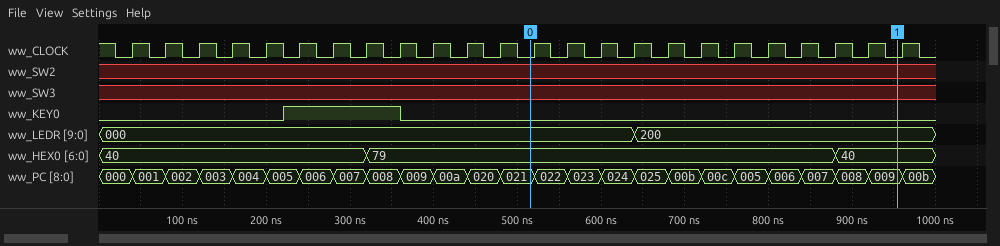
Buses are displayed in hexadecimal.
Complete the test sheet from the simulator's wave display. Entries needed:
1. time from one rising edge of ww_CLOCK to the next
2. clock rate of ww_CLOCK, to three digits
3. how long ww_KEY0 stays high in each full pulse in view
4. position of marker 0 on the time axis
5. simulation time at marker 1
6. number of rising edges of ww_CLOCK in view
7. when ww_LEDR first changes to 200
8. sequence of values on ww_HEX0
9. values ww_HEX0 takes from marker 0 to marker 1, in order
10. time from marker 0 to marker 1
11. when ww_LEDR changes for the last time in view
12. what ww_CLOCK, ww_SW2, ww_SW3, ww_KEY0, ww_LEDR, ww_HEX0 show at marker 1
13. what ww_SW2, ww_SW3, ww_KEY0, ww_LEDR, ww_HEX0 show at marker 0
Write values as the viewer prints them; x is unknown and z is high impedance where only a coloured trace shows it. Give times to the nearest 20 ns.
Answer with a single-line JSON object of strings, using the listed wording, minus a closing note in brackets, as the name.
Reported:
{"time from one rising edge of ww_CLOCK to the next": "40 ns", "clock rate of ww_CLOCK, to three digits": "25.0 MHz", "how long ww_KEY0 stays high in each full pulse in view": "140 ns", "position of marker 0 on the time axis": "520 ns", "simulation time at marker 1": "960 ns", "number of rising edges of ww_CLOCK in view": "24", "when ww_LEDR first changes to 200": "640 ns", "sequence of values on ww_HEX0": "40, 79, 40", "values ww_HEX0 takes from marker 0 to marker 1, in order": "79, 40", "time from marker 0 to marker 1": "440 ns", "when ww_LEDR changes for the last time in view": "640 ns", "what ww_CLOCK, ww_SW2, ww_SW3, ww_KEY0, ww_LEDR, ww_HEX0 show at marker 1": "ww_CLOCK=0, ww_SW2=x, ww_SW3=x, ww_KEY0=0, ww_LEDR=200, ww_HEX0=40", "what ww_SW2, ww_SW3, ww_KEY0, ww_LEDR, ww_HEX0 show at marker 0": "ww_SW2=x, ww_SW3=x, ww_KEY0=0, ww_LEDR=000, ww_HEX0=79"}
